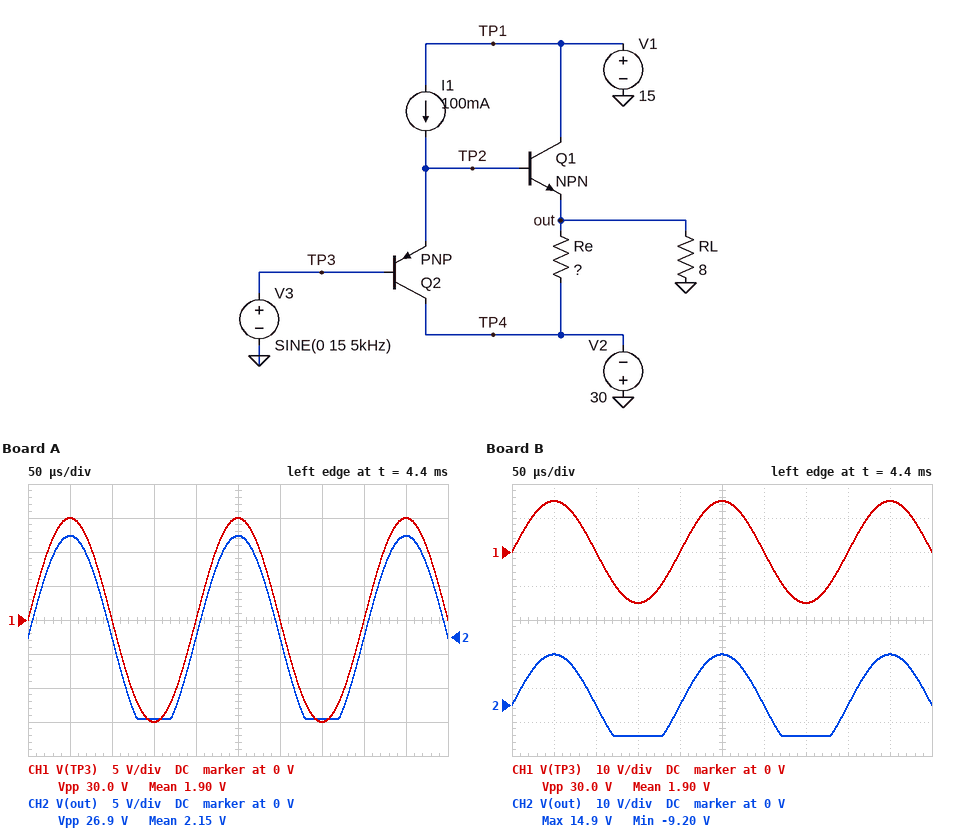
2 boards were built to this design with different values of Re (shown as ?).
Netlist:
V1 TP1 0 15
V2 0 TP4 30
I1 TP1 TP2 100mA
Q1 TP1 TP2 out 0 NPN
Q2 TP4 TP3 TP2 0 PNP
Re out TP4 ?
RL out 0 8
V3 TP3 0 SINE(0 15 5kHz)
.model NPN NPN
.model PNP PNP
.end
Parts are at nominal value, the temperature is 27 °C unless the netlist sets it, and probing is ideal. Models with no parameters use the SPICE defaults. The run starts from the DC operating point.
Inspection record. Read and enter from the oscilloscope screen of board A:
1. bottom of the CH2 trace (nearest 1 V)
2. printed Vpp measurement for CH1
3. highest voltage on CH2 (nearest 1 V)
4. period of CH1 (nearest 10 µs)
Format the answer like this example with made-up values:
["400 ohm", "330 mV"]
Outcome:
["-12 V", "30.0 V", "15 V", "200 µs"]
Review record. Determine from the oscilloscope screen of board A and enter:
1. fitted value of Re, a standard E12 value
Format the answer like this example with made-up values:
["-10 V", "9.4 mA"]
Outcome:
["12 Ω"]
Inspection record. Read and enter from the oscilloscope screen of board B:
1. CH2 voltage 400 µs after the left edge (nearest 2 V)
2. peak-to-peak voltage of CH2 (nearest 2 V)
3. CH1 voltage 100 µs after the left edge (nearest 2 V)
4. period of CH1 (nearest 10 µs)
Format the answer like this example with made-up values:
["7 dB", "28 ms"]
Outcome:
["0 V", "24 V", "0 V", "200 µs"]
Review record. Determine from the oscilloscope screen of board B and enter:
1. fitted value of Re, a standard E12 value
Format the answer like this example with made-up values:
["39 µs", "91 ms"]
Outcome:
["18 Ω"]
